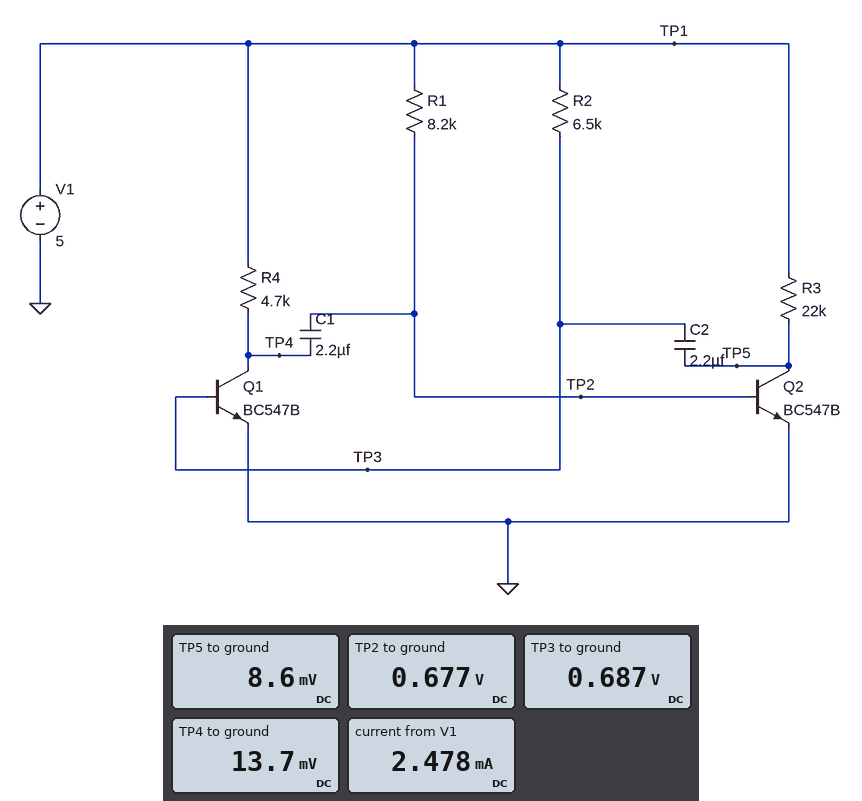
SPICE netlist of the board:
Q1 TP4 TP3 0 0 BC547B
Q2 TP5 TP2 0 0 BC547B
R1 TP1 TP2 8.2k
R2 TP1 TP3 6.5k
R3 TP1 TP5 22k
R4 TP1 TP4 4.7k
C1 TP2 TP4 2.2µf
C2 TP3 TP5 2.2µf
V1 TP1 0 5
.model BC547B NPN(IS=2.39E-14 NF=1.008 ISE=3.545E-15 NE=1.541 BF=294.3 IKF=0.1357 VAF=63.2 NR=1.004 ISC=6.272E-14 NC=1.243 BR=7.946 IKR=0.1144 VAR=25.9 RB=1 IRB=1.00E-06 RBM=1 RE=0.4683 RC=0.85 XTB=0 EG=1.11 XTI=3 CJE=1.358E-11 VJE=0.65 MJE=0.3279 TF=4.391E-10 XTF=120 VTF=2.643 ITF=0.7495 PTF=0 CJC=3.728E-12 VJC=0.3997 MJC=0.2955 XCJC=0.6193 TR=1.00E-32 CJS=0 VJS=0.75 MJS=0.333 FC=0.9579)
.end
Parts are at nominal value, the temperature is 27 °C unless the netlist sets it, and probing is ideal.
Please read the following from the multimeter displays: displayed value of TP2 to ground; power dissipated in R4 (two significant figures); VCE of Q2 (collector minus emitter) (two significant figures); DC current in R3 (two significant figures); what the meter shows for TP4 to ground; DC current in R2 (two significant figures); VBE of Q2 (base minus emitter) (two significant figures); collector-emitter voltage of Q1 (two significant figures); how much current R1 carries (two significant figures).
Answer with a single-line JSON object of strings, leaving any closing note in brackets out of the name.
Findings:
{"displayed value of TP2 to ground": "0.677 V", "power dissipated in R4": "5.3 mW", "VCE of Q2 (collector minus emitter)": "8.6 mV", "DC current in R3": "230 µA", "what the meter shows for TP4 to ground": "13.7 mV", "DC current in R2": "660 µA", "VBE of Q2 (base minus emitter)": "680 mV", "collector-emitter voltage of Q1": "14 mV", "how much current R1 carries": "530 µA"}
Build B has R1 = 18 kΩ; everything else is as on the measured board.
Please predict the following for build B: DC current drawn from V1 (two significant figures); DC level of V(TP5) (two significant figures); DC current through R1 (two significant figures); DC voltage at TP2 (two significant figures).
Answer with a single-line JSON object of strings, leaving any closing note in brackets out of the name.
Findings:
{"DC current drawn from V1": "2.2 mA", "DC level of V(TP5)": "10 mV", "DC current through R1": "240 µA", "DC voltage at TP2": "660 mV"}
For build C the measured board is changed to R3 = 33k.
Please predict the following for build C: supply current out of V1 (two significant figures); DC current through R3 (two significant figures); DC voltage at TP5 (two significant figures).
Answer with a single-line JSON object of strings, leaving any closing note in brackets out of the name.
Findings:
{"supply current out of V1": "2.4 mA", "DC current through R3": "150 µA", "DC voltage at TP5": "8.0 mV"}
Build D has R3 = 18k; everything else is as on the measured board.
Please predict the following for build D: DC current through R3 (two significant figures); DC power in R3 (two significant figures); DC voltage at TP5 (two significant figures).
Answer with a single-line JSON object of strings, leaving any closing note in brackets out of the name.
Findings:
{"DC current through R3": "280 µA", "DC power in R3": "1.4 mW", "DC voltage at TP5": "9.0 mV"}
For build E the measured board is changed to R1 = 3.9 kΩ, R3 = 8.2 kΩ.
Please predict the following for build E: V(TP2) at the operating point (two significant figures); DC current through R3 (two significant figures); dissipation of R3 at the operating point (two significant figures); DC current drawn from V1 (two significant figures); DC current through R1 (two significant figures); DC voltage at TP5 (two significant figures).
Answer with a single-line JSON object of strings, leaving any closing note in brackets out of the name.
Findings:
{"V(TP2) at the operating point": "700 mV", "DC current through R3": "610 µA", "dissipation of R3 at the operating point": "3.0 mW", "DC current drawn from V1": "3.4 mA", "DC current through R1": "1.1 mA", "DC voltage at TP5": "10 mV"}
